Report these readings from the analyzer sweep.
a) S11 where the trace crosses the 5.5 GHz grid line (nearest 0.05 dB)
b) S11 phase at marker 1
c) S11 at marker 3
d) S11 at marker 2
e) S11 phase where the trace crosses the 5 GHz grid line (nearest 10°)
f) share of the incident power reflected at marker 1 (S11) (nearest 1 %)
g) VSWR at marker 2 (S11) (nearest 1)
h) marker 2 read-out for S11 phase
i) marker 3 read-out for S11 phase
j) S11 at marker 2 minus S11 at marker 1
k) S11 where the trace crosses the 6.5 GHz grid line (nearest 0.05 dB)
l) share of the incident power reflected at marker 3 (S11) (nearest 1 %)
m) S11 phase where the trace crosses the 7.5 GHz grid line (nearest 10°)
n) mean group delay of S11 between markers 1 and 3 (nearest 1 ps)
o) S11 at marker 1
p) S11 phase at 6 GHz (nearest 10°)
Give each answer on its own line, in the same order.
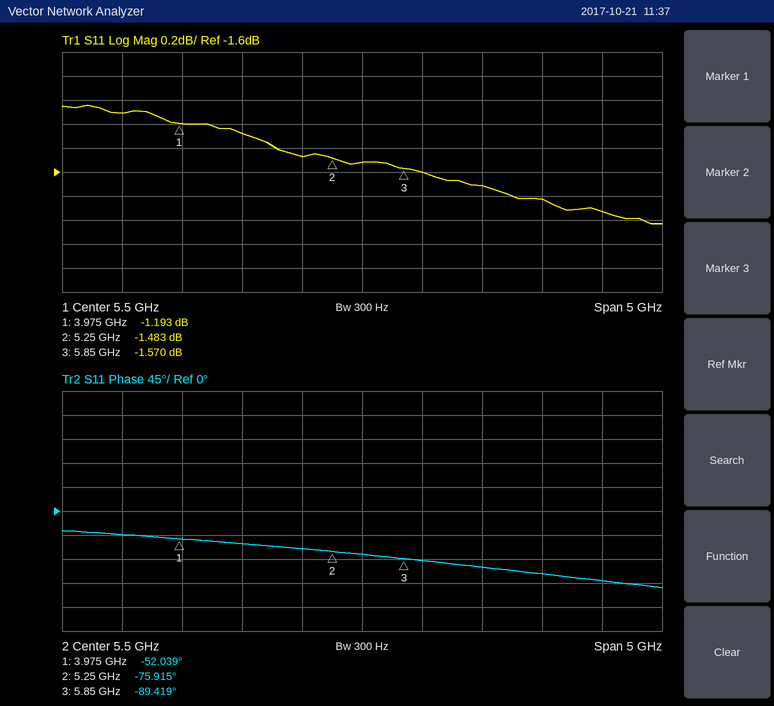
-1.50 dB
-52.039°
-1.570 dB
-1.483 dB
-70°
76 %
12
-75.915°
-89.419°
-0.290 dB
-1.70 dB
70 %
-130°
55 ps
-1.193 dB
-90°
